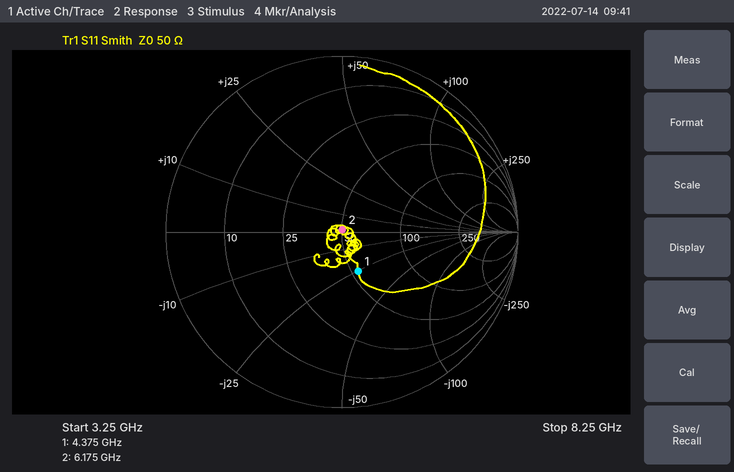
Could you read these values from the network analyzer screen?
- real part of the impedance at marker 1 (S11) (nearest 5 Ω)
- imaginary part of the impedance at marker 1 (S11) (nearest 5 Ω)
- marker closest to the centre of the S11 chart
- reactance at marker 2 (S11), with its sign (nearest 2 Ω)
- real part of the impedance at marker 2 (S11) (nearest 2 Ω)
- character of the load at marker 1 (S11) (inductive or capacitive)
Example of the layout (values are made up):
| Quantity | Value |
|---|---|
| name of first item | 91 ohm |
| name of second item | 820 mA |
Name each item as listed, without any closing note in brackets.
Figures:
| Quantity | Value |
|---|---|
| real part of the impedance at marker 1 (S11) | 55 Ω |
| imaginary part of the impedance at marker 1 (S11) | -25 Ω |
| marker closest to the centre of the S11 chart | marker 2 |
| reactance at marker 2 (S11), with its sign | +2 Ω |
| real part of the impedance at marker 2 (S11) | 50 Ω |
| character of the load at marker 1 (S11) | capacitive |
